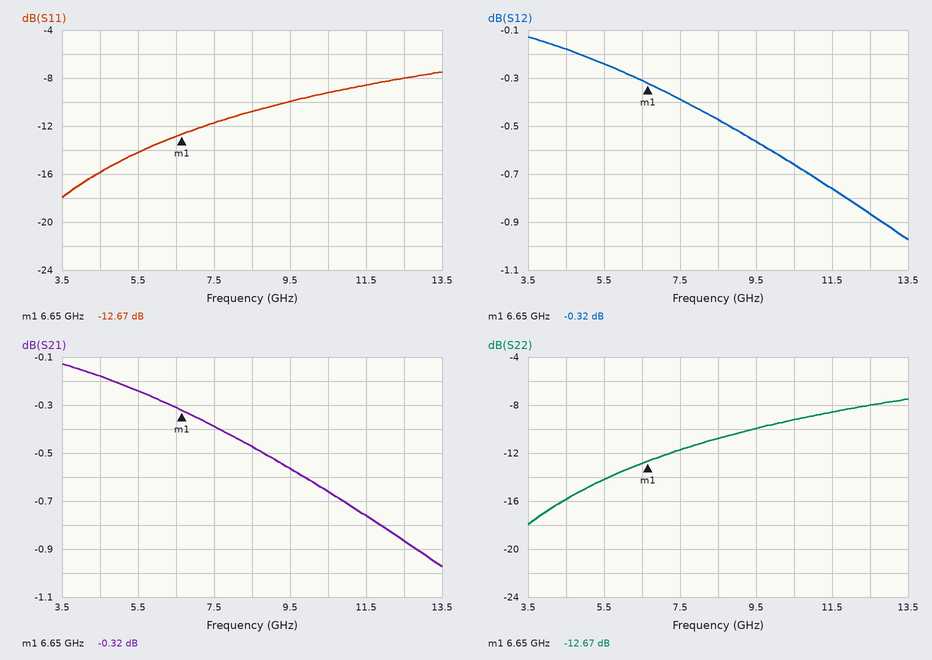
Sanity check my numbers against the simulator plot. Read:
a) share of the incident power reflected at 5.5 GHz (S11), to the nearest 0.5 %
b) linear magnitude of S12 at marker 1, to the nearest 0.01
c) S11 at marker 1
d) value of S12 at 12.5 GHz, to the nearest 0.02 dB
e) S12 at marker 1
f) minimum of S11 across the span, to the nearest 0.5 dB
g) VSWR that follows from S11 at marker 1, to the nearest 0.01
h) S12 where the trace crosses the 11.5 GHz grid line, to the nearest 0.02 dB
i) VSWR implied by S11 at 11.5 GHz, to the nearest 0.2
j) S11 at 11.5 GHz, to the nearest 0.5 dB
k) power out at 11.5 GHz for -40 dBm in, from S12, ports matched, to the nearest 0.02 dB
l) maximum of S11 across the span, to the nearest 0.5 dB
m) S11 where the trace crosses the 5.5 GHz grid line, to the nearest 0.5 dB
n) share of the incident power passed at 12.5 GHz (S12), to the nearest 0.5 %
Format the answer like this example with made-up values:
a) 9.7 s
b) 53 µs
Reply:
a) 4.0 %
b) 0.96
c) -12.67 dB
d) -0.86 dB
e) -0.32 dB
f) -18.0 dB
g) 1.61
h) -0.76 dB
i) 2.2
j) -8.5 dB
k) -40.76 dBm
l) -7.5 dB
m) -14.0 dB
n) 82.0 %
